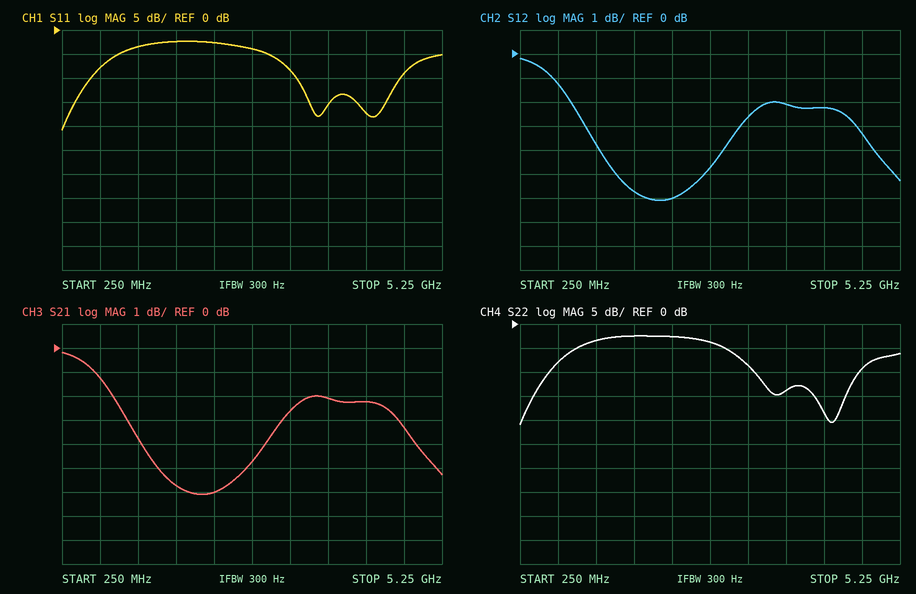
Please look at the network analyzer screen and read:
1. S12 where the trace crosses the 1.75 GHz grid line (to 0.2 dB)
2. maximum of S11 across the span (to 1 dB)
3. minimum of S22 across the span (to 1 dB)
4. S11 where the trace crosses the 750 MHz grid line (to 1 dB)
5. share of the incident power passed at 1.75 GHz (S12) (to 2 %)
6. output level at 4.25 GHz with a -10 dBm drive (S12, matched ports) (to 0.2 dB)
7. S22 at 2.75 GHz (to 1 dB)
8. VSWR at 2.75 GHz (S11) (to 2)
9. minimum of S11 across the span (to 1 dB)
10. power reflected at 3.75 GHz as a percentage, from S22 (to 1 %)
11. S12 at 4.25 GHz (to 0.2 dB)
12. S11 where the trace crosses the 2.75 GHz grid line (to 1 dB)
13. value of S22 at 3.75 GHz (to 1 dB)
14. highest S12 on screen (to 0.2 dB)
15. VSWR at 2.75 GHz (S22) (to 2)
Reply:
-5.8 dB
-2 dB
-21 dB
-8 dB
26 %
-12.2 dBm
-4 dB
4
-21 dB
4 %
-2.2 dB
-4 dB
-14 dB
-0.2 dB
4
